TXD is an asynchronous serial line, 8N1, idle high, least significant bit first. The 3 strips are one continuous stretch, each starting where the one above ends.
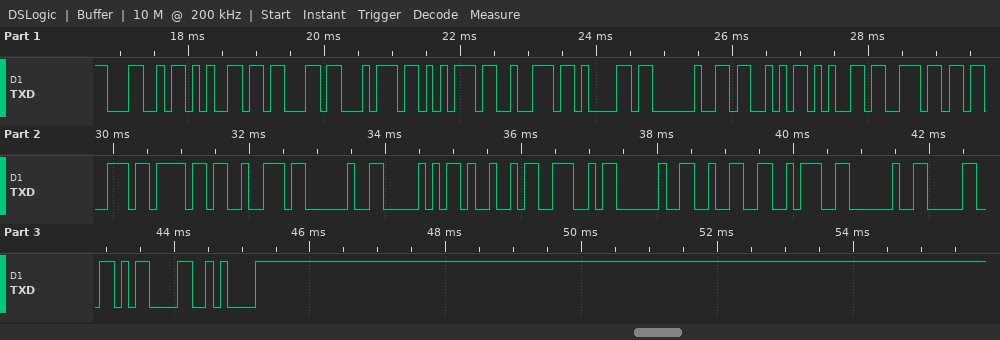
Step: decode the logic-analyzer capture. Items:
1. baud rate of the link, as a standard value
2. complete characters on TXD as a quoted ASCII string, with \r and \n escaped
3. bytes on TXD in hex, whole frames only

9600 baud
"Lectura Sensor PIN 2: 0\r\n"
4C 65 63 74 75 72 61 20 53 65 6E 73 6F 72 20 50 49 4E 20 32 3A 20 30 0D 0A
